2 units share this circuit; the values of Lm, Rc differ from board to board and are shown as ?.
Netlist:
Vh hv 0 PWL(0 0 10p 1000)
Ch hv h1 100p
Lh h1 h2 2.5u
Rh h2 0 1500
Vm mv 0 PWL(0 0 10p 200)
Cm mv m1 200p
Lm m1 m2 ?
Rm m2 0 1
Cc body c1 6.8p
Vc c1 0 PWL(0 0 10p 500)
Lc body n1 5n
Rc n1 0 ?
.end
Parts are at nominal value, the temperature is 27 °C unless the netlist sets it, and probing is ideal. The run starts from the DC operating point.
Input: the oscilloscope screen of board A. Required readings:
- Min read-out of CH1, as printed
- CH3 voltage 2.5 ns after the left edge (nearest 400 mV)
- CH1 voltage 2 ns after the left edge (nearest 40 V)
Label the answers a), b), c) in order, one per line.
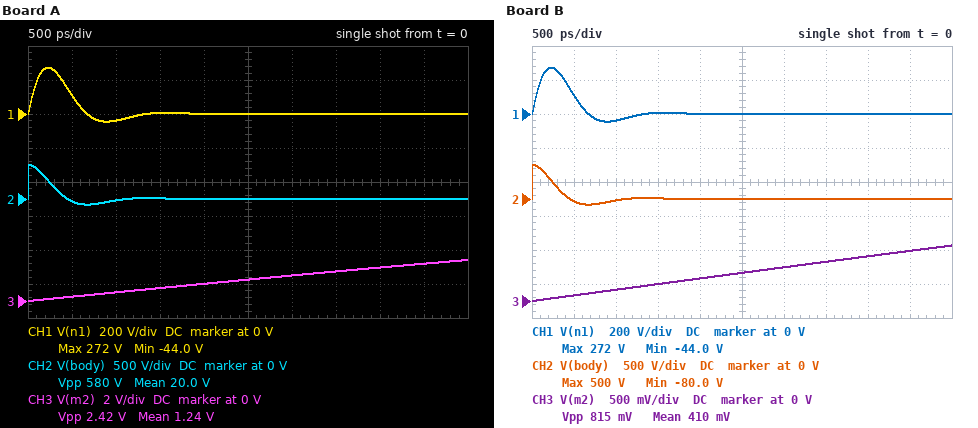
a) -44.0 V
b) 1.2 V
c) 0 V
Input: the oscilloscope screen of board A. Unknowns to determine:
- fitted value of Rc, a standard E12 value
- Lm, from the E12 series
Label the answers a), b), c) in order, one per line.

a) 27 Ω
b) 390 nH
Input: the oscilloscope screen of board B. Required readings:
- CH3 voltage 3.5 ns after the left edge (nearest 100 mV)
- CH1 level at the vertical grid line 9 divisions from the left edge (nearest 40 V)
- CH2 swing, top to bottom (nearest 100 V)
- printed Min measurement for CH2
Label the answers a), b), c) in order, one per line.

a) 600 mV
b) 0 V
c) 600 V
d) -80.0 V
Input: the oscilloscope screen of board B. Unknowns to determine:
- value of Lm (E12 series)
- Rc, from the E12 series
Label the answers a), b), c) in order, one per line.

a) 1.2 µH
b) 27 Ω
